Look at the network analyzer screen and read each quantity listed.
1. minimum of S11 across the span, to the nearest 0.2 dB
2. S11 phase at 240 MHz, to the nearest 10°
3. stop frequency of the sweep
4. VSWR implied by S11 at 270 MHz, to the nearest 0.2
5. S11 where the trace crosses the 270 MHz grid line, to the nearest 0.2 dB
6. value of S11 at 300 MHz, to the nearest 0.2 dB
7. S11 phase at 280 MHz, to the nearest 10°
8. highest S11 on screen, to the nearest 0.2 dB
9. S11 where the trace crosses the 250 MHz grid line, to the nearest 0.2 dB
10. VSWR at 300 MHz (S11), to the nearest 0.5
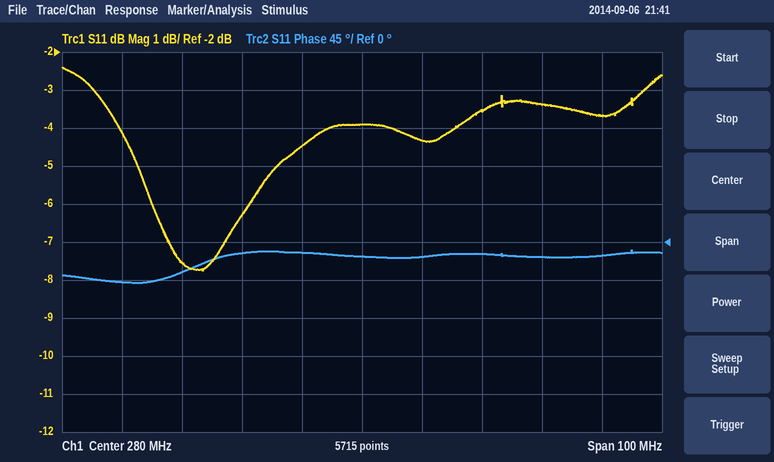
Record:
-7.8 dB
-50°
330 MHz
4.0
-4.4 dB
-3.6 dB
-20°
-2.4 dB
-7.6 dB
5.0
